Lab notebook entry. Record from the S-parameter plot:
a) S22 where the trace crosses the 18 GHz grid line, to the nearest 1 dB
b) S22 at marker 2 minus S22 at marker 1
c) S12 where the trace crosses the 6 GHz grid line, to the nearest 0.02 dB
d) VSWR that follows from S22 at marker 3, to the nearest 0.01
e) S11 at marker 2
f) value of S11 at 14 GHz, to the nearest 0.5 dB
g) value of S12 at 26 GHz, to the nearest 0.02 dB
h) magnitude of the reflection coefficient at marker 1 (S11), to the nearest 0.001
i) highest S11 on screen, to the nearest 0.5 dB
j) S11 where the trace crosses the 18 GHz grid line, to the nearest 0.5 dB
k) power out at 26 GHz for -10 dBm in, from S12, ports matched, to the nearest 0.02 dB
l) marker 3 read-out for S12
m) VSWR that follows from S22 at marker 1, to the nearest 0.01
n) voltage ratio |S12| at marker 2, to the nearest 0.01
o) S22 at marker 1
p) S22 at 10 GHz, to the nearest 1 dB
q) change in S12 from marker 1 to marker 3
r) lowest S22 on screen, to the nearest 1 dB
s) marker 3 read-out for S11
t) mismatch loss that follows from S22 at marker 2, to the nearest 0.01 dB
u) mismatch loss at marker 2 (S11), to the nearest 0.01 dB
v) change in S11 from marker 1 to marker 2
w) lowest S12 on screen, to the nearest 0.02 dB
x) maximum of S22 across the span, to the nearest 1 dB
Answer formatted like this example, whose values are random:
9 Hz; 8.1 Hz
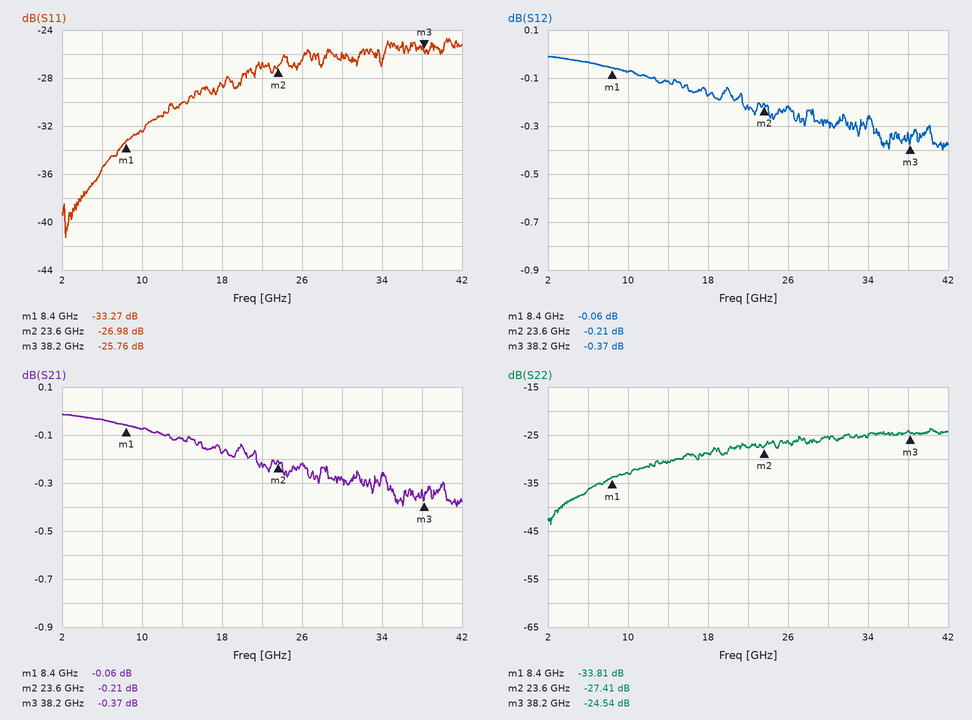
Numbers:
-29 dB; 6.40 dB; -0.04 dB; 1.13; -26.98 dB; -30.0 dB; -0.22 dB; 0.022; -24.5 dB; -28.5 dB; -10.22 dBm; -0.37 dB; 1.04; 0.98; -33.81 dB; -33 dB; -0.31 dB; -44 dB; -25.76 dB; 0.01 dB; 0.01 dB; 6.29 dB; -0.40 dB; -24 dB
